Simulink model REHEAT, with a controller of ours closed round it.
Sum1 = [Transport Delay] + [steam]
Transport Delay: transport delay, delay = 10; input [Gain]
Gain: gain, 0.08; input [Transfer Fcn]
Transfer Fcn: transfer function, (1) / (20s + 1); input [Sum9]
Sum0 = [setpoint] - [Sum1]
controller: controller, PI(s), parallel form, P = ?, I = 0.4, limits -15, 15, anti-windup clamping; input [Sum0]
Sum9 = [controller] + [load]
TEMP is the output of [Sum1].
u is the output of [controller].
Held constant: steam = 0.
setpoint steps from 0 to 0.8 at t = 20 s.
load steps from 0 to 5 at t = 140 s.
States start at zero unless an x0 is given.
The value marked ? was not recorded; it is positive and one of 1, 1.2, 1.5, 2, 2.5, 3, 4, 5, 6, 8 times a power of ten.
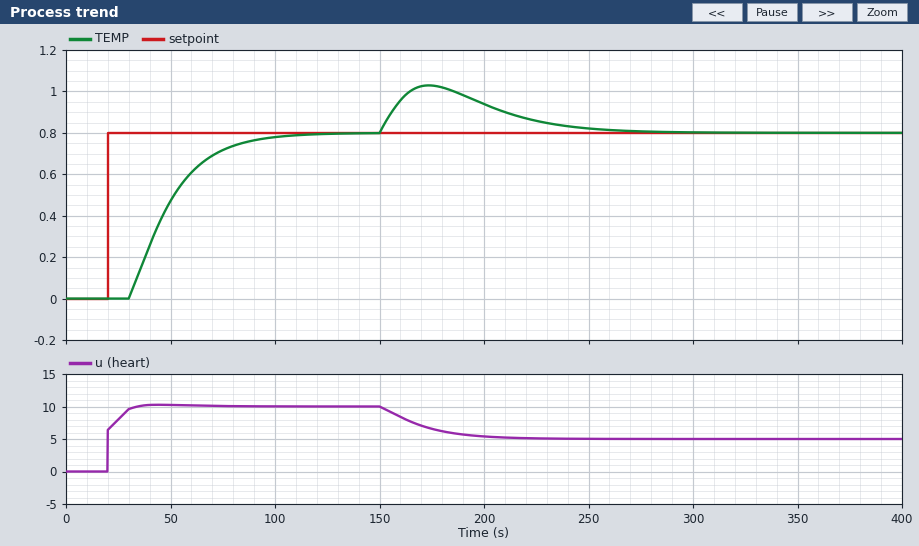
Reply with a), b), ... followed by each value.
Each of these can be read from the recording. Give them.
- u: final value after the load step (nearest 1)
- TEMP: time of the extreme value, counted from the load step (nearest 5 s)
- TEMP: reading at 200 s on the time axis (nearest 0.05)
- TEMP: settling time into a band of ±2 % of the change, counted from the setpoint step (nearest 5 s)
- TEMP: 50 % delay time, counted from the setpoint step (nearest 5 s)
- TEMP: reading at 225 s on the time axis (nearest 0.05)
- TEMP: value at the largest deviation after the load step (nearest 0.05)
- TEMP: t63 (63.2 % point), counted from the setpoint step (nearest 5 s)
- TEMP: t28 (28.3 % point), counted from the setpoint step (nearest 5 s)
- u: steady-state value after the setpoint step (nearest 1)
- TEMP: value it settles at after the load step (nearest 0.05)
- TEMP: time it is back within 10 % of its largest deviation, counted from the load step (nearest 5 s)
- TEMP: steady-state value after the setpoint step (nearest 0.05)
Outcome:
a) 5
b) 35 s
c) 0.95
d) 85 s
e) 25 s
f) 0.85
g) 1.05
h) 30 s
i) 20 s
j) 10
k) 0.80
l) 110 s
m) 0.80
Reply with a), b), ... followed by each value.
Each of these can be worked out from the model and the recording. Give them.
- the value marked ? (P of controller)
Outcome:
a) 8
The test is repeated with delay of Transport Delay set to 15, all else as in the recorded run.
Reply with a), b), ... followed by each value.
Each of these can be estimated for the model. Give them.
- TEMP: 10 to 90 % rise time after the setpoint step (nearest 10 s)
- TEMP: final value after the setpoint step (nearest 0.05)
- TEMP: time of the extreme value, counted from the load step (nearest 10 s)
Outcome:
a) 30 s
b) 0.80
c) 40 s
